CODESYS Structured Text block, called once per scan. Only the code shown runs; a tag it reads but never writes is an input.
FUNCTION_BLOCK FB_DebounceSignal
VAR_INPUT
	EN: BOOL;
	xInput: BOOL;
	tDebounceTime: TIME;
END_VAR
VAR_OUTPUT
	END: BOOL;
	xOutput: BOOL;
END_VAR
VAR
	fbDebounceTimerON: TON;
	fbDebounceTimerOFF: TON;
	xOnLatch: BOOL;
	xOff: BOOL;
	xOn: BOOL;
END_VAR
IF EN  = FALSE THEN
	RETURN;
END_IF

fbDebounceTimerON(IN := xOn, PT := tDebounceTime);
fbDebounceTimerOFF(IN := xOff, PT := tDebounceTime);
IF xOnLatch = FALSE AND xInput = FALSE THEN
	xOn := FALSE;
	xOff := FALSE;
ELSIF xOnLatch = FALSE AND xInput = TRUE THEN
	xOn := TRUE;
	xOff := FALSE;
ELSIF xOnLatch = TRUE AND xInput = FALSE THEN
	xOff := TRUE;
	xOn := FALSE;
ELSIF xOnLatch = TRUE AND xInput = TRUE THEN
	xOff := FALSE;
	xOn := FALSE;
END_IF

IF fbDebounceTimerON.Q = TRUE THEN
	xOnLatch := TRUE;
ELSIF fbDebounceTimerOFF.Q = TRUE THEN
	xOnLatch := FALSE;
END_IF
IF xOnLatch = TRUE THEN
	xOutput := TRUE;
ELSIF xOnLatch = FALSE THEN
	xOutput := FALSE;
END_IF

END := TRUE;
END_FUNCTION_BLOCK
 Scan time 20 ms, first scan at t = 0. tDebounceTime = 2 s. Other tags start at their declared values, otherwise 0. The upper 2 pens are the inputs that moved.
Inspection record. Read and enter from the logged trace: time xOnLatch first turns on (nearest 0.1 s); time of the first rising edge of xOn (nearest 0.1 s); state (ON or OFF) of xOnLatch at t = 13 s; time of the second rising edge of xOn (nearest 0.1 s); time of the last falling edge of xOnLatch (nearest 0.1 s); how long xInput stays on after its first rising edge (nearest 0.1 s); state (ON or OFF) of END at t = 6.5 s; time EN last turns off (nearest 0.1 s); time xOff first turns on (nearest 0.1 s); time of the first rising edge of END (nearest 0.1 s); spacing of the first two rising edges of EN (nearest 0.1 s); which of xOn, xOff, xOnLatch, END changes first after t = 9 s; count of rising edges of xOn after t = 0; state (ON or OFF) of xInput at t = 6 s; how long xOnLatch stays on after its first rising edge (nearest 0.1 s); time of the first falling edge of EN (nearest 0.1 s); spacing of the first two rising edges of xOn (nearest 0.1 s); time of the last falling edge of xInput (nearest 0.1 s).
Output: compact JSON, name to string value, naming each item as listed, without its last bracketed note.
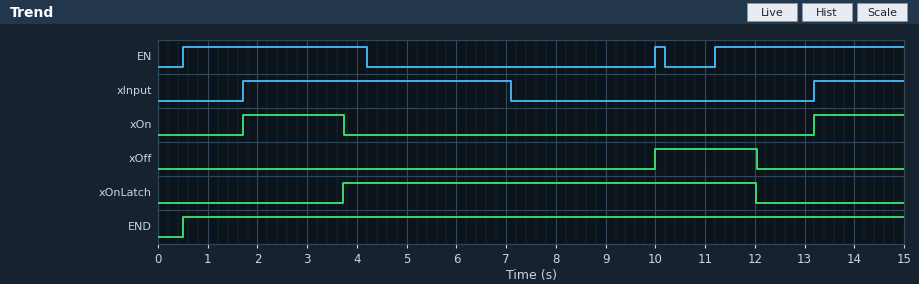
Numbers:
{"time xOnLatch first turns on": "3.7 s", "time of the first rising edge of xOn": "1.7 s", "state (ON or OFF) of xOnLatch at t = 13 s": "OFF", "time of the second rising edge of xOn": "13.2 s", "time of the last falling edge of xOnLatch": "12.0 s", "how long xInput stays on after its first rising edge": "5.4 s", "state (ON or OFF) of END at t = 6.5 s": "ON", "time EN last turns off": "10.2 s", "time xOff first turns on": "10.0 s", "time of the first rising edge of END": "0.5 s", "spacing of the first two rising edges of EN": "9.5 s", "which of xOn, xOff, xOnLatch, END changes first after t = 9 s": "xOff", "count of rising edges of xOn after t = 0": "2", "state (ON or OFF) of xInput at t = 6 s": "ON", "how long xOnLatch stays on after its first rising edge": "8.3 s", "time of the first falling edge of EN": "4.2 s", "spacing of the first two rising edges of xOn": "11.5 s", "time of the last falling edge of xInput": "7.1 s"}
